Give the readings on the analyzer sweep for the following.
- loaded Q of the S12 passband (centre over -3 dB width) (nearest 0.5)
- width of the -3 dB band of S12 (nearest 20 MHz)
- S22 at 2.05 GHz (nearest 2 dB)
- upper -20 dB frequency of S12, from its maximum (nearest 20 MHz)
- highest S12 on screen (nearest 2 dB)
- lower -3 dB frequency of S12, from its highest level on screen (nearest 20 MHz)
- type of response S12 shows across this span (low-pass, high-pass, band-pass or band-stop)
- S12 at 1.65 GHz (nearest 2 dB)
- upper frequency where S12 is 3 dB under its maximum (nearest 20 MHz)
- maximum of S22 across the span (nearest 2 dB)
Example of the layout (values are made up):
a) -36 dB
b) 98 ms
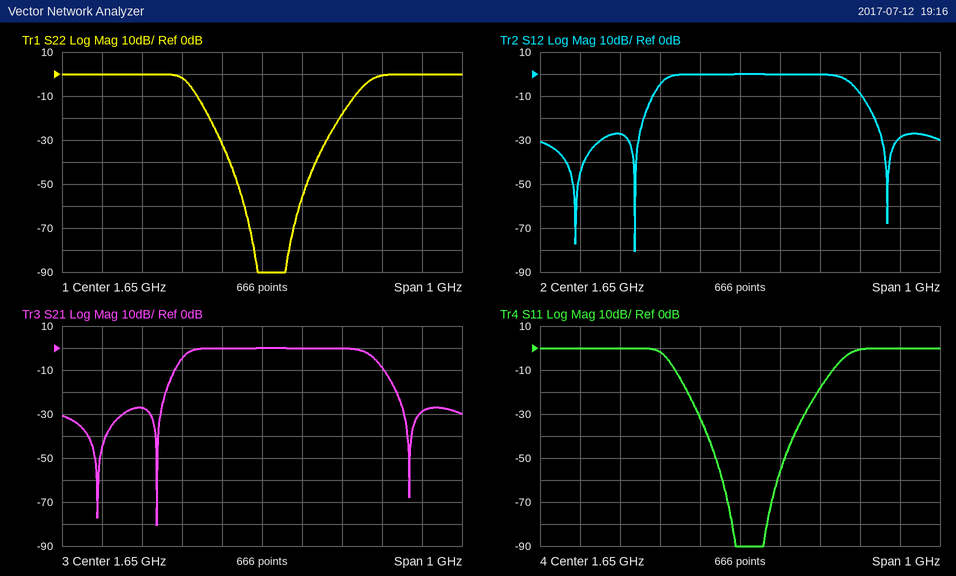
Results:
a) 3.5
b) 460 MHz
c) 0 dB
d) 1.98 GHz
e) 0 dB
f) 1.46 GHz
g) band-pass
h) 0 dB
i) 1.92 GHz
j) 0 dB
